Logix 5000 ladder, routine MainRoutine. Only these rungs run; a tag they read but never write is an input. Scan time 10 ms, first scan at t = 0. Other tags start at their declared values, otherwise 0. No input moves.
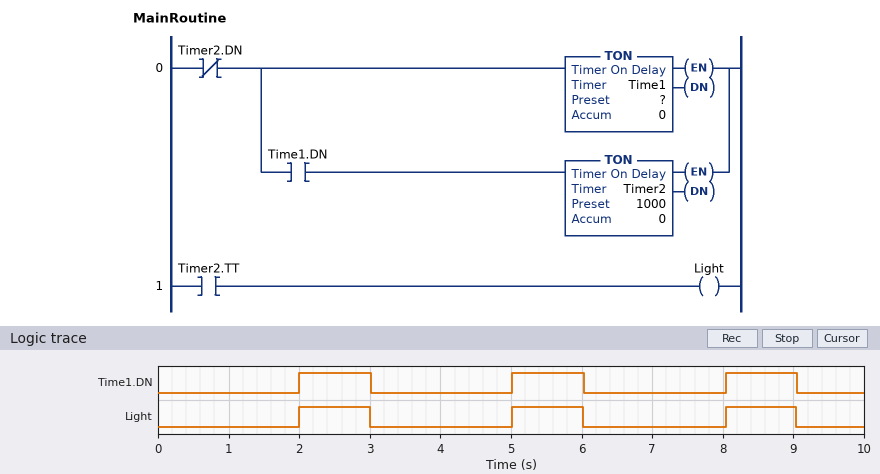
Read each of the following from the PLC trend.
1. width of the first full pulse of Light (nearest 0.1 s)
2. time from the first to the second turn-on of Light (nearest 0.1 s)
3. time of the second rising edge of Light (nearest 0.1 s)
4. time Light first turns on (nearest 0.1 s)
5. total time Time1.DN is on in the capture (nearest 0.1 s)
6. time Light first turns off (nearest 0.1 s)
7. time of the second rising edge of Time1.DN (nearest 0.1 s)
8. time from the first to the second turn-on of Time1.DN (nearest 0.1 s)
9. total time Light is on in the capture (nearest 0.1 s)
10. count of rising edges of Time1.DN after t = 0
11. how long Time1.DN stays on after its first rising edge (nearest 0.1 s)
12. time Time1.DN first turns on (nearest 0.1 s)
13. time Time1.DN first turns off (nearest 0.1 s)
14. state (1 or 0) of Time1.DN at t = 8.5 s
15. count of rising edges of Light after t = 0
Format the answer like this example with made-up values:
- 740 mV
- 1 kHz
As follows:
- 1.0 s
- 3.0 s
- 5.0 s
- 2.0 s
- 3.0 s
- 3.0 s
- 5.0 s
- 3.0 s
- 3.0 s
- 3
- 1.0 s
- 2.0 s
- 3.0 s
- 1
- 3
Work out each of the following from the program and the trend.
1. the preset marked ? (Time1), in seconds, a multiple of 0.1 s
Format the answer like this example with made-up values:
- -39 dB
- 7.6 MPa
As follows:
- 2.0 s
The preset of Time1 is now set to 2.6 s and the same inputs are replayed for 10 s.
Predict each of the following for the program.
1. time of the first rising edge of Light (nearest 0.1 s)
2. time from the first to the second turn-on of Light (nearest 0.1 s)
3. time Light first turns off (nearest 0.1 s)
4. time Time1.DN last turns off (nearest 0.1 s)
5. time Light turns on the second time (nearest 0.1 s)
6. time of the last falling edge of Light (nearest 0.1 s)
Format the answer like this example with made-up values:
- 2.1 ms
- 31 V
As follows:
- 2.6 s
- 3.6 s
- 3.6 s
- 7.2 s
- 6.2 s
- 7.2 s
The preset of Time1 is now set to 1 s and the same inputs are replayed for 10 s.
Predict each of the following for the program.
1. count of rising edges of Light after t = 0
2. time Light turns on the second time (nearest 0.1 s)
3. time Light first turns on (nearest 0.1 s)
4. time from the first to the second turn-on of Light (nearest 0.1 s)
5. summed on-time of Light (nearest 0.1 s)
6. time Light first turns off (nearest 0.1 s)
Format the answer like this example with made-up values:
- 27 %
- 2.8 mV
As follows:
- 5
- 3.0 s
- 1.0 s
- 2.0 s
- 4.9 s
- 2.0 s
